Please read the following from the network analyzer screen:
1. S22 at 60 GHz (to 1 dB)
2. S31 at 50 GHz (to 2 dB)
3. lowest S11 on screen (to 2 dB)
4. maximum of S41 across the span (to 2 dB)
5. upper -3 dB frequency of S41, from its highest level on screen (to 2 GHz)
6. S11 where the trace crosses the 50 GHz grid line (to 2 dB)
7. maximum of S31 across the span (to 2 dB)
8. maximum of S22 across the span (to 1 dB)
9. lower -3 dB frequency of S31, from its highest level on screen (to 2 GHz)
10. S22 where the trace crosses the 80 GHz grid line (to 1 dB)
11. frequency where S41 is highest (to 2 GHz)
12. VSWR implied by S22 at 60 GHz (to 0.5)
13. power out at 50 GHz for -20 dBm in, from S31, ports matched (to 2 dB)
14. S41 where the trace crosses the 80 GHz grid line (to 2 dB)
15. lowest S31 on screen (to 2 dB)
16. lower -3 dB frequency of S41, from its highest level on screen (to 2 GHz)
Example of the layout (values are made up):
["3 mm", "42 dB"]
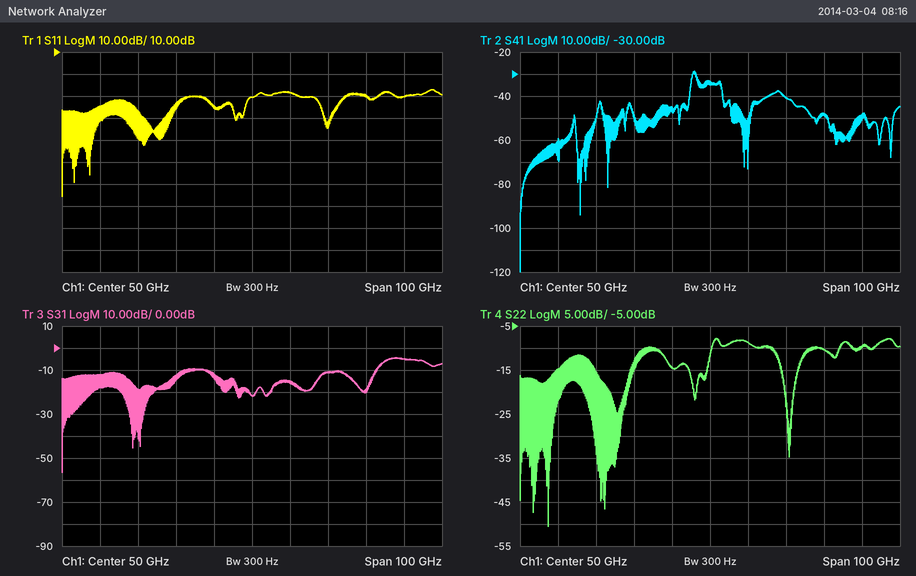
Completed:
["-9 dB", "-22 dB", "-56 dB", "-28 dB", "46 GHz", "-10 dB", "-4 dB", "-8 dB", "84 GHz", "-10 dB", "46 GHz", "2.0", "-42 dBm", "-48 dB", "-56 dB", "46 GHz"]
